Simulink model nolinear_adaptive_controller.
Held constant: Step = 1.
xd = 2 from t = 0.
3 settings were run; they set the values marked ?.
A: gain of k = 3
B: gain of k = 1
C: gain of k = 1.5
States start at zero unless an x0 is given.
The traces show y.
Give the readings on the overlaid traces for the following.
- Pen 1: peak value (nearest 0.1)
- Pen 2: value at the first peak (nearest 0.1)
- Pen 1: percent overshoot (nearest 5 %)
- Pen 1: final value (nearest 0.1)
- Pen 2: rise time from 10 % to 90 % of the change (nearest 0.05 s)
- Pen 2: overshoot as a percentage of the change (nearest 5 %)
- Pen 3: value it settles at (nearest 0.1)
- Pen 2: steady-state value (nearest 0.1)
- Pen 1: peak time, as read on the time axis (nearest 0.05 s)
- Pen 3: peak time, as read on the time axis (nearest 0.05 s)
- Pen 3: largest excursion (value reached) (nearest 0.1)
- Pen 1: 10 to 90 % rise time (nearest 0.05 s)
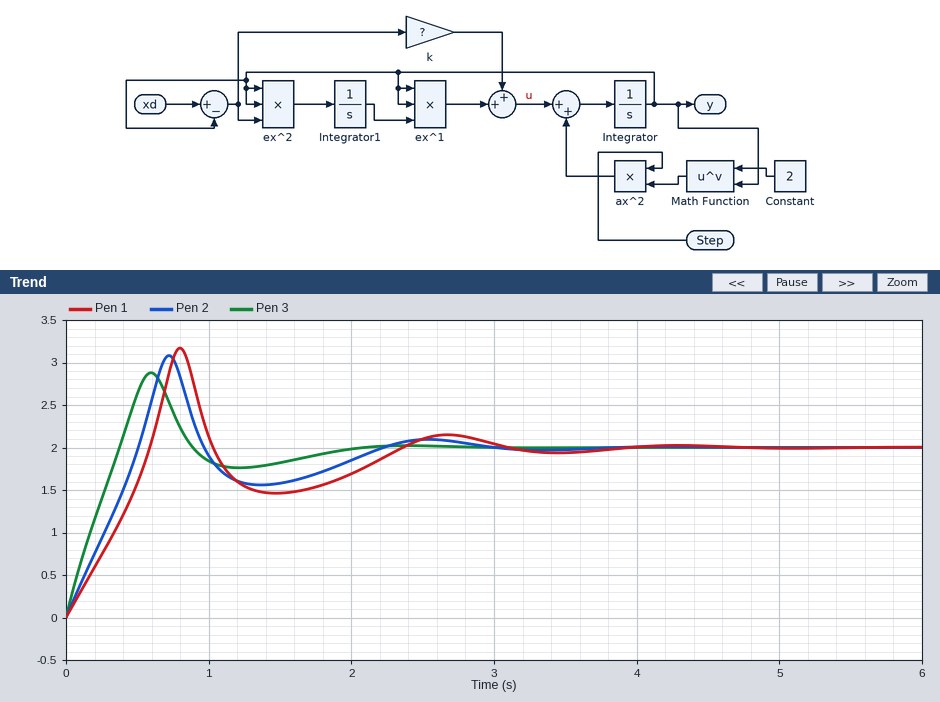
3.2
3.1
60 %
2.0
0.40 s
55 %
2.0
2.0
0.80 s
0.60 s
2.9
0.50 s
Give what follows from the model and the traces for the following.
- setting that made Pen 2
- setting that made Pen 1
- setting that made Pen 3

C
B
A
